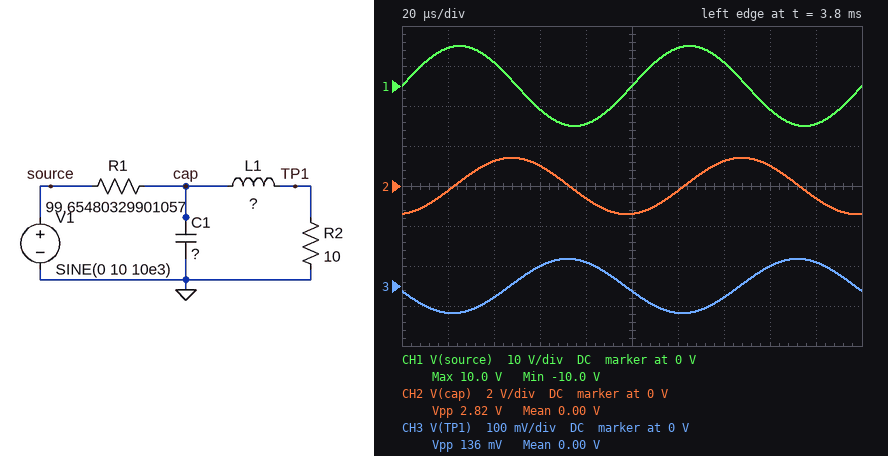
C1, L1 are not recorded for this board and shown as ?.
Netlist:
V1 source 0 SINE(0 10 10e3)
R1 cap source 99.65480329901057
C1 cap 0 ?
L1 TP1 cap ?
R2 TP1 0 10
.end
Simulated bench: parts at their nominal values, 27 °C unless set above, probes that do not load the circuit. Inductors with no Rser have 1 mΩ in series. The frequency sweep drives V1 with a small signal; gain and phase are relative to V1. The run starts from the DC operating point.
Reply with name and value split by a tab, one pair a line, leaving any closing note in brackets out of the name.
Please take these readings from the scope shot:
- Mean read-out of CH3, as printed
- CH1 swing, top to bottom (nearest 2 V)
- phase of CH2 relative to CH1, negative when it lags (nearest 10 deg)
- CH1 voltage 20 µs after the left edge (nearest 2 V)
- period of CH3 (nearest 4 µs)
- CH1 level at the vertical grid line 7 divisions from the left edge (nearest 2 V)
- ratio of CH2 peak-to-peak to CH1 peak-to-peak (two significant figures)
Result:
Mean read-out of CH3, as printed	0.00 V
CH1 swing, top to bottom	20 V
phase of CH2 relative to CH1, negative when it lags	-80 deg
CH1 voltage 20 µs after the left edge	10 V
period of CH3	100 µs
CH1 level at the vertical grid line 7 divisions from the left edge	6 V
ratio of CH2 peak-to-peak to CH1 peak-to-peak	0.14
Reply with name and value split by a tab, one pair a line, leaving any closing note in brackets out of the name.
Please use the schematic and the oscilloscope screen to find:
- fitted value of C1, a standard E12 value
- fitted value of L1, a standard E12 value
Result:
fitted value of C1, a standard E12 value	1.2 µF
fitted value of L1, a standard E12 value	3.3 mH
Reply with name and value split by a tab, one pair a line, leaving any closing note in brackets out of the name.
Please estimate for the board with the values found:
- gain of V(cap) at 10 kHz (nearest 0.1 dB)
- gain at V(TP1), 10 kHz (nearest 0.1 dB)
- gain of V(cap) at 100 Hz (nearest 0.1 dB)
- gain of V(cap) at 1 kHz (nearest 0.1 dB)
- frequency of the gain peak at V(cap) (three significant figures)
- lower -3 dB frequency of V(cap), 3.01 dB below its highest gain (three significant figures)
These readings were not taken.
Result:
gain of V(cap) at 10 kHz	-17.0 dB
gain at V(TP1), 10 kHz	-43.4 dB
gain of V(cap) at 100 Hz	-20.6 dB
gain of V(cap) at 1 kHz	-12.6 dB
frequency of the gain peak at V(cap)	2.64 kHz
lower -3 dB frequency of V(cap), 3.01 dB below its highest gain	1.88 kHz
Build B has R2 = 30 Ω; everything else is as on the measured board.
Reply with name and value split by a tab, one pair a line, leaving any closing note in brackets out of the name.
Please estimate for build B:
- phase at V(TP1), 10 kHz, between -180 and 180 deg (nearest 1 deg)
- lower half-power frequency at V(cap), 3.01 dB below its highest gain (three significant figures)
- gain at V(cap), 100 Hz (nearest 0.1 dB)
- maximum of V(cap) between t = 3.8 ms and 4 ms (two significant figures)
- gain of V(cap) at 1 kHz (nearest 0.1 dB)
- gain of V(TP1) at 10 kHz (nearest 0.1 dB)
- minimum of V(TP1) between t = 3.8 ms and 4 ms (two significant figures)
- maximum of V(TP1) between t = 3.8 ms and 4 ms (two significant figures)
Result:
phase at V(TP1), 10 kHz, between -180 and 180 deg	-163 deg
lower half-power frequency at V(cap), 3.01 dB below its highest gain	1.52 kHz
gain at V(cap), 100 Hz	-12.7 dB
maximum of V(cap) between t = 3.8 ms and 4 ms	1.4 V
gain of V(cap) at 1 kHz	-10.5 dB
gain of V(TP1) at 10 kHz	-33.9 dB
minimum of V(TP1) between t = 3.8 ms and 4 ms	-200 mV
maximum of V(TP1) between t = 3.8 ms and 4 ms	200 mV
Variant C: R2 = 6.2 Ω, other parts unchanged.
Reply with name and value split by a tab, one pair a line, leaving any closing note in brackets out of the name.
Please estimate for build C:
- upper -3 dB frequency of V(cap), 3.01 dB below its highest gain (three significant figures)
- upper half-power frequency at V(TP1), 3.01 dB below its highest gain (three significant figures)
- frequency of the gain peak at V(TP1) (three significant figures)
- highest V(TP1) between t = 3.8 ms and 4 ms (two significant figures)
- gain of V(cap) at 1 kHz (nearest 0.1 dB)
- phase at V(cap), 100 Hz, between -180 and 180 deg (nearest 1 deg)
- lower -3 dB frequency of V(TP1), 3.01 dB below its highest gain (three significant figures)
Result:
upper -3 dB frequency of V(cap), 3.01 dB below its highest gain	3.54 kHz
upper half-power frequency at V(TP1), 3.01 dB below its highest gain	3.08 kHz
frequency of the gain peak at V(TP1)	2.34 kHz
highest V(TP1) between t = 3.8 ms and 4 ms	42 mV
gain of V(cap) at 1 kHz	-12.7 dB
phase at V(cap), 100 Hz, between -180 and 180 deg	17 deg
lower -3 dB frequency of V(TP1), 3.01 dB below its highest gain	1.20 kHz
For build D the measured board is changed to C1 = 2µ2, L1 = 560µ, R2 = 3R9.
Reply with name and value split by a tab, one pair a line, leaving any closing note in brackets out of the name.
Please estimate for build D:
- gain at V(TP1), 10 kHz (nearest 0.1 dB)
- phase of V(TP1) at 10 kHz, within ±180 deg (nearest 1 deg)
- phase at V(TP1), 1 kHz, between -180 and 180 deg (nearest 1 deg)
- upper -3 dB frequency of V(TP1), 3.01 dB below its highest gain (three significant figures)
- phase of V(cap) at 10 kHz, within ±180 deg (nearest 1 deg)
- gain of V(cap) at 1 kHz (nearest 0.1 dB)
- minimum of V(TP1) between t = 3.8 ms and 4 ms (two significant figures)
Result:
gain at V(TP1), 10 kHz	-40.0 dB
phase of V(TP1) at 10 kHz, within ±180 deg	-167 deg
phase at V(TP1), 1 kHz, between -180 and 180 deg	-5 deg
upper -3 dB frequency of V(TP1), 3.01 dB below its highest gain	5.29 kHz
phase of V(cap) at 10 kHz, within ±180 deg	-83 deg
gain of V(cap) at 1 kHz	-25.5 dB
minimum of V(TP1) between t = 3.8 ms and 4 ms	-100 mV
